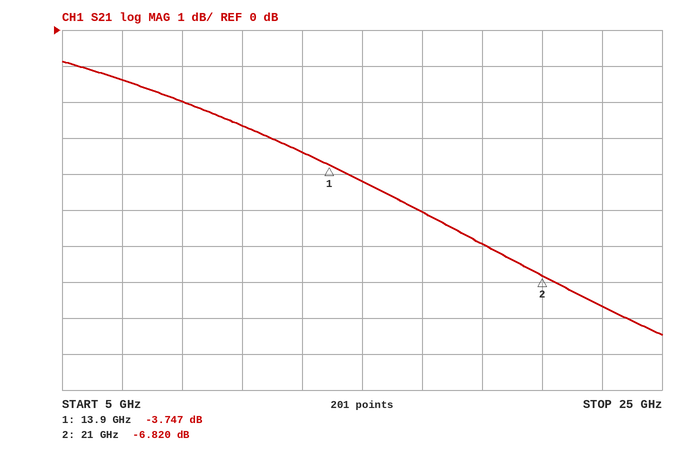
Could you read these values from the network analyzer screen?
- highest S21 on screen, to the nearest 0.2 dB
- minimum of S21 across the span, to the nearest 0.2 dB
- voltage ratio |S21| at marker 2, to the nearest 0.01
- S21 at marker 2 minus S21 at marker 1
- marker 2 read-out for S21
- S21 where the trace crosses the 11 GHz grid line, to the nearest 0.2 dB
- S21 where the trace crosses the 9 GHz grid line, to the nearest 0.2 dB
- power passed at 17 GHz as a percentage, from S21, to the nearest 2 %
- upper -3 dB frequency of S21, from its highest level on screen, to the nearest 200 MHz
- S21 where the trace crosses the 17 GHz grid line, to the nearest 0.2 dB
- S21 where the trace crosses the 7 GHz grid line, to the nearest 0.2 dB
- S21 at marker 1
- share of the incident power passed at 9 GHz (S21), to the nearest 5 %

-0.8 dB
-8.4 dB
0.46
-3.073 dB
-6.820 dB
-2.6 dB
-2.0 dB
32 %
14.2 GHz
-5.0 dB
-1.4 dB
-3.747 dB
65 %
